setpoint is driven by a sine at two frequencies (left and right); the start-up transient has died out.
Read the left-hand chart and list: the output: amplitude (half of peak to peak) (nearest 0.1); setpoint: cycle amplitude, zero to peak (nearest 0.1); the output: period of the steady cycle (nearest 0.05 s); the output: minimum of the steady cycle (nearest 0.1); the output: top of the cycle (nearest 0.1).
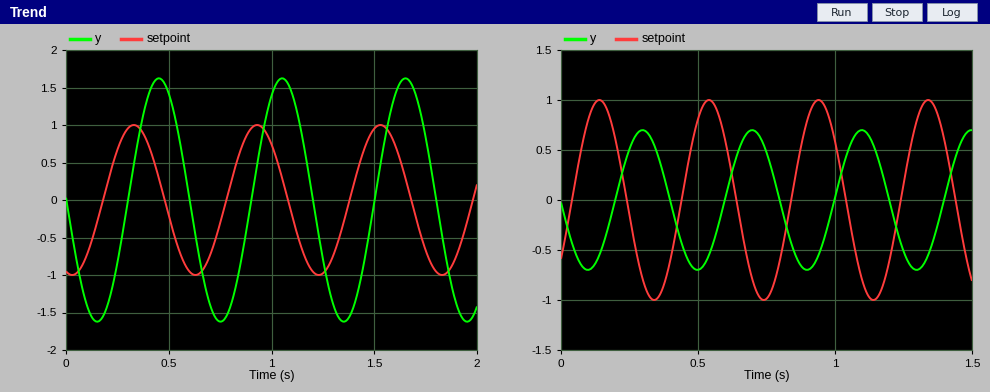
1.6
1.0
0.60 s
-1.6
1.6
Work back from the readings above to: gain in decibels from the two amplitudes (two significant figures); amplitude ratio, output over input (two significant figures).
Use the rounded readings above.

4.1 dB
1.6
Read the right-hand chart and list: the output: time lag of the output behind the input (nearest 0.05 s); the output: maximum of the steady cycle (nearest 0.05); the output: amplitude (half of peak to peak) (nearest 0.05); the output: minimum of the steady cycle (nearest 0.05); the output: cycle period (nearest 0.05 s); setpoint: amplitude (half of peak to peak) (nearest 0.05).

0.15 s
0.70
0.70
-0.70
0.40 s
1.00
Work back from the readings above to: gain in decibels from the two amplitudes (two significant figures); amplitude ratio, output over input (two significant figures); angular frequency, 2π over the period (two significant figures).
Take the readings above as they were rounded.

-3.1 dB
0.70
16 rad/s
